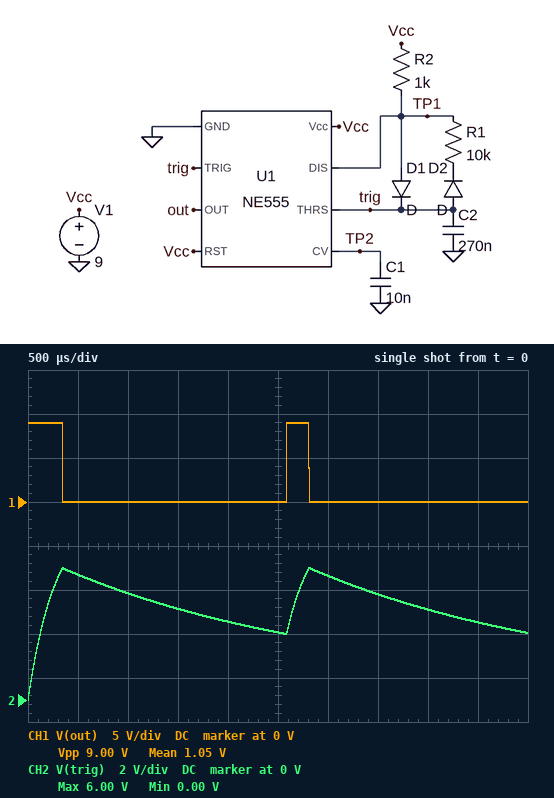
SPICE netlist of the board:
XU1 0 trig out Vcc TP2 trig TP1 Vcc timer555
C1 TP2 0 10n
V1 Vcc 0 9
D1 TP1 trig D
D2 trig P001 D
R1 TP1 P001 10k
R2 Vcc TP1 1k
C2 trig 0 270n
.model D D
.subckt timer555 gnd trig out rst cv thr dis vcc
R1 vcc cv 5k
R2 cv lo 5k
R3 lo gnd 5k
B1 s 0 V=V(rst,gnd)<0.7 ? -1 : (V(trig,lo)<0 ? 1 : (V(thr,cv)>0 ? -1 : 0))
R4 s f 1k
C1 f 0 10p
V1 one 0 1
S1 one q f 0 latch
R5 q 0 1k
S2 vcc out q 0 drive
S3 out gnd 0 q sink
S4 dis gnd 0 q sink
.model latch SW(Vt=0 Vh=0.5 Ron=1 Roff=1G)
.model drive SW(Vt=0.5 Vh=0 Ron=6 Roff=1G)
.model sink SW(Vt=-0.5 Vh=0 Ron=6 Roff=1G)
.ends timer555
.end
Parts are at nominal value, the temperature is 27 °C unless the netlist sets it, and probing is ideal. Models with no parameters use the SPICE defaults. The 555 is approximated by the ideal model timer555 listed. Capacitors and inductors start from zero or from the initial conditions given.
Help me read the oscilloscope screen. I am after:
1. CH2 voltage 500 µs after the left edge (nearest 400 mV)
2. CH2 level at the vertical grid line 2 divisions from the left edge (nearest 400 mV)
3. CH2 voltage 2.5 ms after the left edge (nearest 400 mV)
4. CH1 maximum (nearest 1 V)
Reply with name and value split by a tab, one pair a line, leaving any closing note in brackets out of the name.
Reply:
CH2 voltage 500 µs after the left edge	5.6 V
CH2 level at the vertical grid line 2 divisions from the left edge	4.8 V
CH2 voltage 2.5 ms after the left edge	3.2 V
CH1 maximum	9 V
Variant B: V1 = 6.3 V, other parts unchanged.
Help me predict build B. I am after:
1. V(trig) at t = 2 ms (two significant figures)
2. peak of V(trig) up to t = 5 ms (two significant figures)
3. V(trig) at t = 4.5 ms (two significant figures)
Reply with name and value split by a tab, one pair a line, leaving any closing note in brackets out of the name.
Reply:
V(trig) at t = 2 ms	2.6 V
peak of V(trig) up to t = 5 ms	4.2 V
V(trig) at t = 4.5 ms	2.7 V
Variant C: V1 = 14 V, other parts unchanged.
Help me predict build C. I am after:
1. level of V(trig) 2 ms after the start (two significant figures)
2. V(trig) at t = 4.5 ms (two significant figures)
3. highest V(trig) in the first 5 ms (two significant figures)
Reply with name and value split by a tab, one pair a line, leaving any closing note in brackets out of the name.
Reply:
level of V(trig) 2 ms after the start	5.4 V
V(trig) at t = 4.5 ms	5.1 V
highest V(trig) in the first 5 ms	9.3 V
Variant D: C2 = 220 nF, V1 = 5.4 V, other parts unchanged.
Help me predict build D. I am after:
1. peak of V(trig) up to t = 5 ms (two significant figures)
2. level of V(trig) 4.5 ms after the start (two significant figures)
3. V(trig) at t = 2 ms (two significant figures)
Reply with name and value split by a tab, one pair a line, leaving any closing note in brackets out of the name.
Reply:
peak of V(trig) up to t = 5 ms	3.6 V
level of V(trig) 4.5 ms after the start	1.9 V
V(trig) at t = 2 ms	2.0 V
